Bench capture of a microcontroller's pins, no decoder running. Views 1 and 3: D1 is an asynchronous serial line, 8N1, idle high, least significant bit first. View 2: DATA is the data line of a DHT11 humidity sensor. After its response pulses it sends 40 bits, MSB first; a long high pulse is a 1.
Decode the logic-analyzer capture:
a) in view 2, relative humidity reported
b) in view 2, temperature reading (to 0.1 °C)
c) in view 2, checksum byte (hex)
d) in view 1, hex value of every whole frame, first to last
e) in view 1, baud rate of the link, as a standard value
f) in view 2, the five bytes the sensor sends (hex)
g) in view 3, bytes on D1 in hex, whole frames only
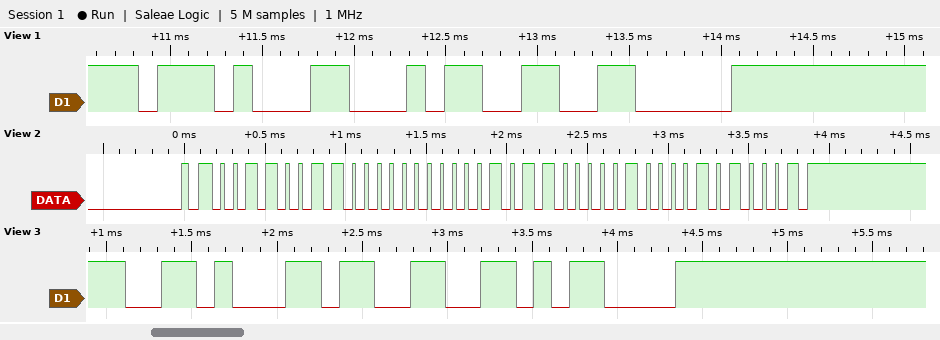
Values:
51 %
22.8 °C
0x51
17 34 06
9600 baud
33 00 16 08 51
16 33 0D
